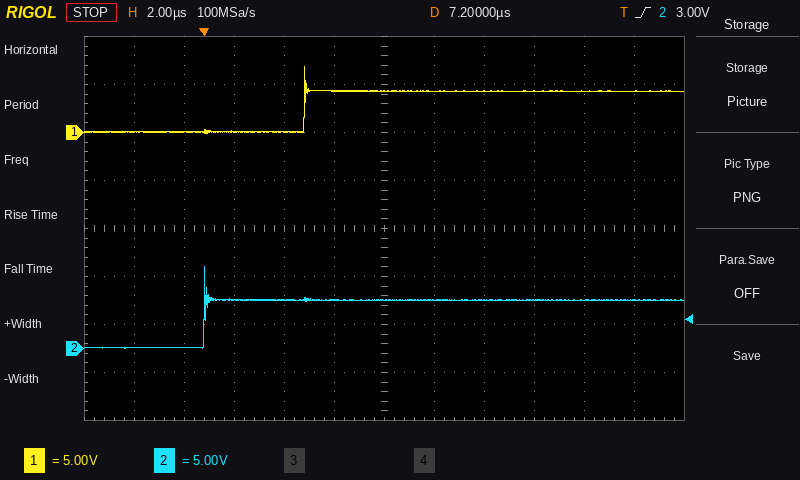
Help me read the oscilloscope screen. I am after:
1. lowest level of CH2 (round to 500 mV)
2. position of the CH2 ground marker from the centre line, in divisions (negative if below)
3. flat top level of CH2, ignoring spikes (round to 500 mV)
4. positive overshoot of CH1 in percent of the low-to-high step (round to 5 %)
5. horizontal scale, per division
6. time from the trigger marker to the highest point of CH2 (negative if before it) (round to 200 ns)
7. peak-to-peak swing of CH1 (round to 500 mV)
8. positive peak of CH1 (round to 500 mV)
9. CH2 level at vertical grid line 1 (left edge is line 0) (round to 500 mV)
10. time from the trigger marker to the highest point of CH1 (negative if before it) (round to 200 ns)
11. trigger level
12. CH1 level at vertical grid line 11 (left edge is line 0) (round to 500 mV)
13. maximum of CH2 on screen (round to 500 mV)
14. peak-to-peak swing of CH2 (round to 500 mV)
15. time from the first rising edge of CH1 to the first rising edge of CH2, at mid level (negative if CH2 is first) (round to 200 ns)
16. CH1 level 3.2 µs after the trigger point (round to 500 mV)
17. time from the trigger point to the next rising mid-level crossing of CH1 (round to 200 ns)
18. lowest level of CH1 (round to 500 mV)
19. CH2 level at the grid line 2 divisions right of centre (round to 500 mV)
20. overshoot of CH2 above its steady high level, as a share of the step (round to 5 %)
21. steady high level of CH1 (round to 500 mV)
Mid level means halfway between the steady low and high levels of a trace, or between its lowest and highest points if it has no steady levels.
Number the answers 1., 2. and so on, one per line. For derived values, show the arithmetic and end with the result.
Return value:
1. 0.0 V
2. -2.5 div
3. 5.0 V
4. 60 %
5. 2 µs
6. 0.0 µs
7. 7.0 V − (0.0 V) = 7.0 V
8. 7.0 V
9. 0.0 V
10. +4.0 µs
11. 3.00 V
12. 4.5 V
13. 8.5 V
14. 8.5 V − (0.0 V) = 8.5 V
15. -4.0 µs
16. 0.0 V
17. 4.0 µs
18. 0.0 V
19. 5.0 V
20. 70 %
21. 4.5 V
